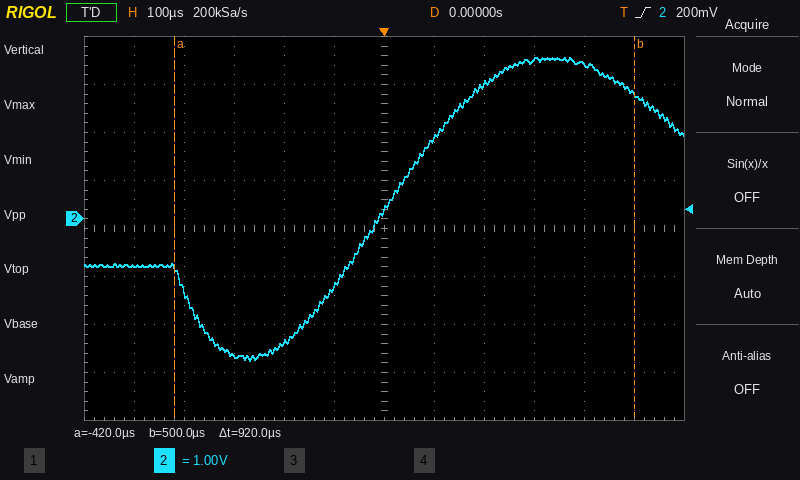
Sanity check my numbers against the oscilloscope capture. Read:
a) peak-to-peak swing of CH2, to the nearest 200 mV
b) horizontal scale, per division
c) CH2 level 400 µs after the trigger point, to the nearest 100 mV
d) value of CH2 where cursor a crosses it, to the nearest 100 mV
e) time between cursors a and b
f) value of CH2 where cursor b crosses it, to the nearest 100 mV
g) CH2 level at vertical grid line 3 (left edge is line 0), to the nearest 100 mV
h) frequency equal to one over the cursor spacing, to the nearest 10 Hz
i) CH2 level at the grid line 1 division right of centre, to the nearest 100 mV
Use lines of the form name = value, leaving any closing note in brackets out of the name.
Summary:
peak-to-peak swing of CH2, to the nearest 200 mV = 6.4 V
horizontal scale, per division = 100 µs
CH2 level 400 µs after the trigger point, to the nearest 100 mV = 3.2 V
value of CH2 where cursor a crosses it, to the nearest 100 mV = -1.0 V
time between cursors a and b = 920 µs
value of CH2 where cursor b crosses it, to the nearest 100 mV = 2.6 V
CH2 level at vertical grid line 3 (left edge is line 0), to the nearest 100 mV = -2.8 V
frequency equal to one over the cursor spacing, to the nearest 10 Hz = 1.09 kHz
CH2 level at the grid line 1 division right of centre, to the nearest 100 mV = 1.7 V
